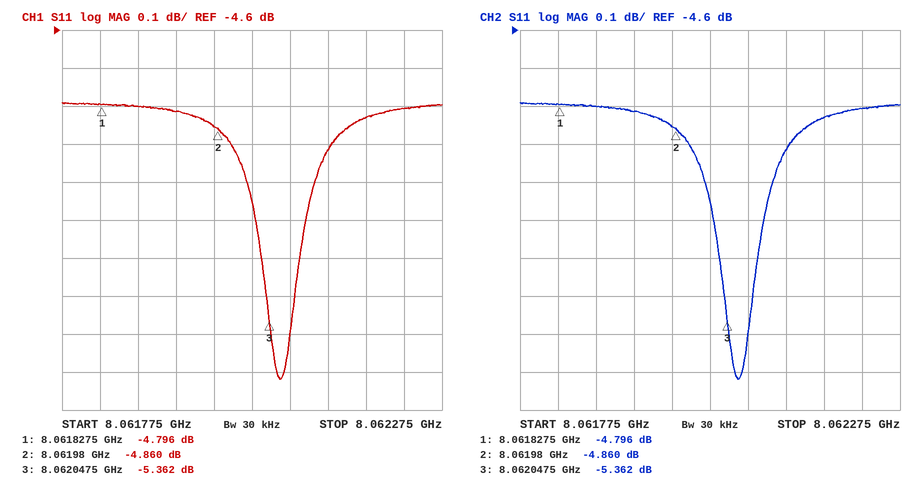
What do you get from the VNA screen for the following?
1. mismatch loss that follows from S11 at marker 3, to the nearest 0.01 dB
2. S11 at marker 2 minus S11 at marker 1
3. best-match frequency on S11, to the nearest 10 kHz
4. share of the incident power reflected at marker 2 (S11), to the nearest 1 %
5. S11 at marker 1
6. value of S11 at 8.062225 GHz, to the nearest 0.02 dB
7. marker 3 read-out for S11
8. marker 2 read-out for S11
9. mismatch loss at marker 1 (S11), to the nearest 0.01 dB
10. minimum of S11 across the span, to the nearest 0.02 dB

1.49 dB
-0.064 dB
8.06206 GHz
33 %
-4.796 dB
-4.80 dB
-5.362 dB
-4.860 dB
1.75 dB
-5.52 dB
